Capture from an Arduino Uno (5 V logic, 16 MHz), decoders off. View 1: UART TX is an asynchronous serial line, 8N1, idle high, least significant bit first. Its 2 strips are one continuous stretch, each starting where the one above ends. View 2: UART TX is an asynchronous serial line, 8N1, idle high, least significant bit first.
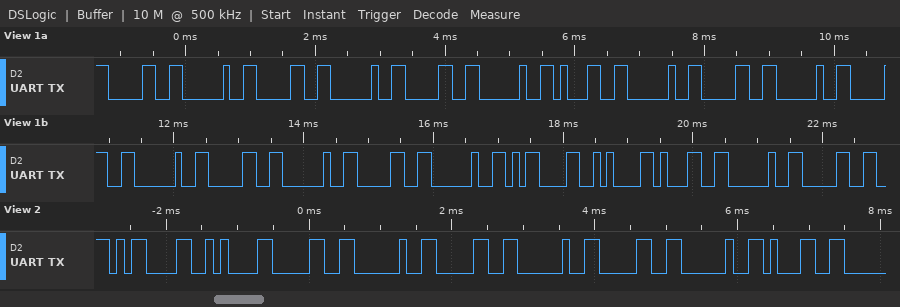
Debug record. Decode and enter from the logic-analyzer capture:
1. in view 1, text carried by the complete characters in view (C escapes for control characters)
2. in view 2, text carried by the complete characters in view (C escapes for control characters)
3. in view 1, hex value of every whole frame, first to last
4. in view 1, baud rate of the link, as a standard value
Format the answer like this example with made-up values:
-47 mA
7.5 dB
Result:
"0 0 0 1 0 0 0 0 \r\n1 0"
"\r\n0 0 0 1"
0x30 0x20 0x30 0x20 0x30 0x20 0x31 0x20 0x30 0x20 0x30 0x20 0x30 0x20 0x30 0x20 0x0D 0x0A 0x31 0x20 0x30
9600 baud
